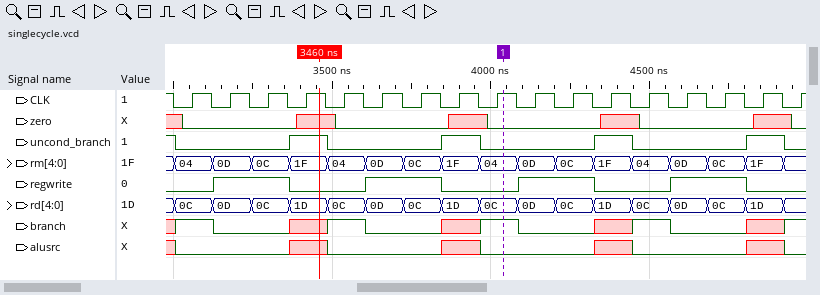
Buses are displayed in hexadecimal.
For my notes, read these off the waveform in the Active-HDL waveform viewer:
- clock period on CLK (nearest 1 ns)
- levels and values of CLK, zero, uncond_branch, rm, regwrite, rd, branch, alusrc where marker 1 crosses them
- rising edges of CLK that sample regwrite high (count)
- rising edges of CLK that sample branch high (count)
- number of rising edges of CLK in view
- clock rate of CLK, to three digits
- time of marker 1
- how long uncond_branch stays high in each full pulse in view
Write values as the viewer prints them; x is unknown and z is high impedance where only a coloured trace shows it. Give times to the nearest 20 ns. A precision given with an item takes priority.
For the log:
120 ns
CLK=1, zero=0, uncond_branch=0, rm=04, regwrite=0, rd=0C, branch=1, alusrc=0
8
5
17
8.33 MHz
4040 ns
120 ns, 120 ns, 120 ns, 120 ns
